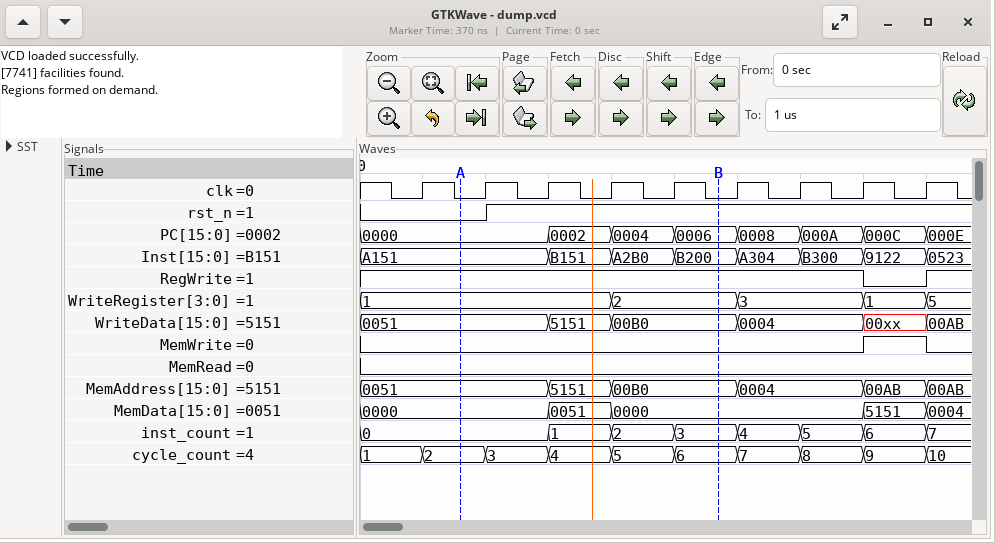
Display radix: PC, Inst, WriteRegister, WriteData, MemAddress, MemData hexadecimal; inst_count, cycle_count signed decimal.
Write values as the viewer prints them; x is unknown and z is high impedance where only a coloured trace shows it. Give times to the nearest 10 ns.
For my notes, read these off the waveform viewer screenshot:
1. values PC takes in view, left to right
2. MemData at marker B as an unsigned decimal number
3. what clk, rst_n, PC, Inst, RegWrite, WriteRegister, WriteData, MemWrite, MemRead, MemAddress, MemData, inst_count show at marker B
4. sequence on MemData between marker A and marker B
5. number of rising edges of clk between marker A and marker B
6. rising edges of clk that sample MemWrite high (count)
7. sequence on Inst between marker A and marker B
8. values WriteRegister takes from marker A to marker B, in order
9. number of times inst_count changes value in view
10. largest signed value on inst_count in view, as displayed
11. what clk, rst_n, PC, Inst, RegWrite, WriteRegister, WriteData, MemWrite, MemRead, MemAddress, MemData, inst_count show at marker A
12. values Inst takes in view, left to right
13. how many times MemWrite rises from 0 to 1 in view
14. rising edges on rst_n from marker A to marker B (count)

0000, 0002, 0004, 0006, 0008, 000A, 000C, 000E
0
clk=0, rst_n=1, PC=0006, Inst=B200, RegWrite=1, WriteRegister=2, WriteData=00B0, MemWrite=0, MemRead=0, MemAddress=00B0, MemData=0000, inst_count=3
0000, 0051, 0000
4
1
A151, B151, A2B0, B200
1, 2
7
7
clk=0, rst_n=0, PC=0000, Inst=A151, RegWrite=1, WriteRegister=1, WriteData=0051, MemWrite=0, MemRead=0, MemAddress=0051, MemData=0000, inst_count=0
A151, B151, A2B0, B200, A304, B300, 9122, 0523
1
1
